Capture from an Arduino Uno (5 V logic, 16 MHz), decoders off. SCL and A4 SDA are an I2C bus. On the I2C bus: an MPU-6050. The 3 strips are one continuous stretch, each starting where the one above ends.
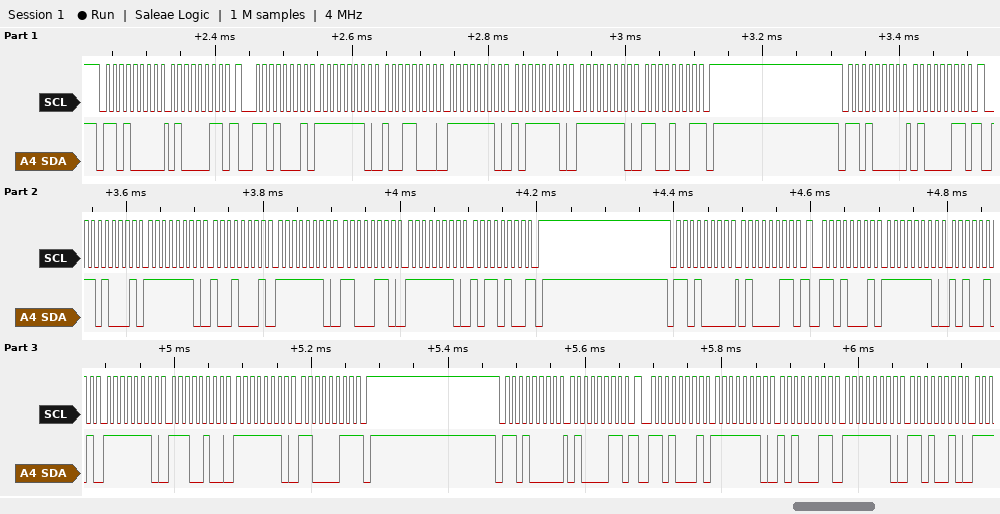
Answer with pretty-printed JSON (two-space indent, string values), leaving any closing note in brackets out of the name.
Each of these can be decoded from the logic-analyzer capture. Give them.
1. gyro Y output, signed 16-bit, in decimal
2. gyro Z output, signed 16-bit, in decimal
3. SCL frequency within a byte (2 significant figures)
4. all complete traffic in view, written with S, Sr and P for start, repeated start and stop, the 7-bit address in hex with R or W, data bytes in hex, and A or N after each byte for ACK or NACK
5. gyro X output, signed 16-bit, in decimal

{
  "gyro Y output, signed 16-bit, in decimal": "-322",
  "gyro Z output, signed 16-bit, in decimal": "-311",
  "SCL frequency within a byte": "100 kHz",
  "all complete traffic in view, written with S, Sr and P for start, repeated start and stop, the 7-bit address in hex with R or W, data bytes in hex, and A or N after each byte for ACK or NACK": "S 68W A 43 A Sr 68R A FE A 98 A FE A BE A FE A C9 N P S 68W A 43 A Sr 68R A FE A 91 A FE A C6 A FE A B4 N P S 68W A 43 A Sr 68R A FE A A5 A FE A E4 A FE A C3 N P S 68W A 43 A Sr 68R A FE A A3 A FE A D2 A",
  "gyro X output, signed 16-bit, in decimal": "-360"
}
